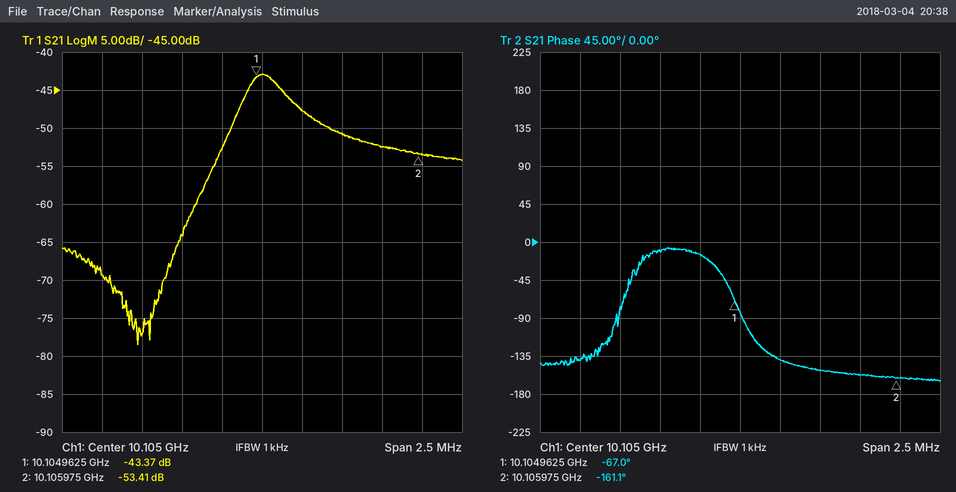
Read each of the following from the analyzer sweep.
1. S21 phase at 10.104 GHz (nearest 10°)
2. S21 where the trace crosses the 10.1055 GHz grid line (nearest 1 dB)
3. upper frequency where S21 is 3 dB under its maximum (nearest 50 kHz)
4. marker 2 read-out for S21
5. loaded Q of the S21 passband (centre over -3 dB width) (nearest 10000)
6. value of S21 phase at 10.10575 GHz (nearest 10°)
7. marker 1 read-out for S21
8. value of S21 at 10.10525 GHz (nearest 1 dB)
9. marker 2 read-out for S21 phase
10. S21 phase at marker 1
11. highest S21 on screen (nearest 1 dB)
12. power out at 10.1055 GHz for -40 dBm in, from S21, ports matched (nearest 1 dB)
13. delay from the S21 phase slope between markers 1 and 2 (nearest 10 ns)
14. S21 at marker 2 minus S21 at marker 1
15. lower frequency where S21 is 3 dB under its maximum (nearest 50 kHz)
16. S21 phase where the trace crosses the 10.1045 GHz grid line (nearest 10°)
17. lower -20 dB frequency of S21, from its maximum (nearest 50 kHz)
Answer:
-140°
-51 dB
10.10515 GHz
-53.41 dB
40000
-160°
-43.37 dB
-48 dB
-161.1°
-67.0°
-43 dB
-91 dBm
260 ns
-10.04 dB
10.10490 GHz
-10°
10.10450 GHz
